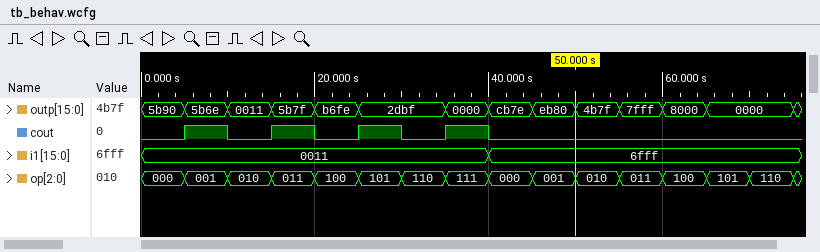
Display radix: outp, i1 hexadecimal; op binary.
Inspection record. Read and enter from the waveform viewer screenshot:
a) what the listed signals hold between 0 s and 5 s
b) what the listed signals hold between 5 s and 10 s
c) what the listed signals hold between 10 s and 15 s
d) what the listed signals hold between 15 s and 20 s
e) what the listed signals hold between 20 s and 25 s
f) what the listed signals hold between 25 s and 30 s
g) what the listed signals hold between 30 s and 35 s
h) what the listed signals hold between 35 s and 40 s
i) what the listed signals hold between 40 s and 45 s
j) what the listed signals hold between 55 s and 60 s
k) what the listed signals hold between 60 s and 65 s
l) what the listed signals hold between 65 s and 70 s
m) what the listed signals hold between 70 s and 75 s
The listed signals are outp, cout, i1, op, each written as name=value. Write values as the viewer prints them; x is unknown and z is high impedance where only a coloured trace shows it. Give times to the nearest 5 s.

outp=5b90, cout=0, i1=0011, op=000
outp=5b6e, cout=1, i1=0011, op=001
outp=0011, cout=0, i1=0011, op=010
outp=5b7f, cout=1, i1=0011, op=011
outp=b6fe, cout=0, i1=0011, op=100
outp=2dbf, cout=1, i1=0011, op=101
outp=2dbf, cout=0, i1=0011, op=110
outp=0000, cout=1, i1=0011, op=111
outp=cb7e, cout=0, i1=6fff, op=000
outp=7fff, cout=0, i1=6fff, op=011
outp=8000, cout=0, i1=6fff, op=100
outp=0000, cout=0, i1=6fff, op=101
outp=0000, cout=0, i1=6fff, op=110
